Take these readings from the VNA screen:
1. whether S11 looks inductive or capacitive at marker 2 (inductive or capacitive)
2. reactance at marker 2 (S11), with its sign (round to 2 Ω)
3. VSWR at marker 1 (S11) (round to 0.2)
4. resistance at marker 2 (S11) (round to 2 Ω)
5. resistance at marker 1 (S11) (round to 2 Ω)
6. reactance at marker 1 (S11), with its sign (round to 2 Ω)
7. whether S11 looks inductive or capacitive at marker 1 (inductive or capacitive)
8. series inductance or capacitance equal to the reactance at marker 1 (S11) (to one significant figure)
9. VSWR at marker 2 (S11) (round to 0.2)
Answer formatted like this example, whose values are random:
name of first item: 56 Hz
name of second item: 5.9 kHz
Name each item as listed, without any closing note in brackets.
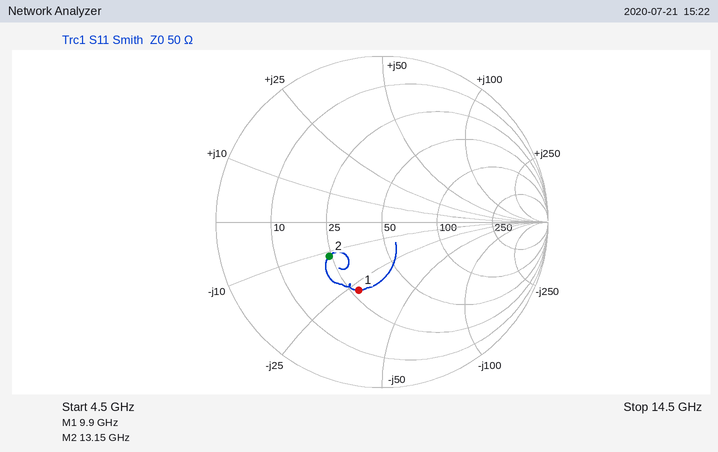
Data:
whether S11 looks inductive or capacitive at marker 2: capacitive
reactance at marker 2 (S11), with its sign: -12 Ω
VSWR at marker 1 (S11): 2.6
resistance at marker 2 (S11): 24 Ω
resistance at marker 1 (S11): 28 Ω
reactance at marker 1 (S11), with its sign: -28 Ω
whether S11 looks inductive or capacitive at marker 1: capacitive
series inductance or capacitance equal to the reactance at marker 1 (S11): 600 fF
VSWR at marker 2 (S11): 2.2
